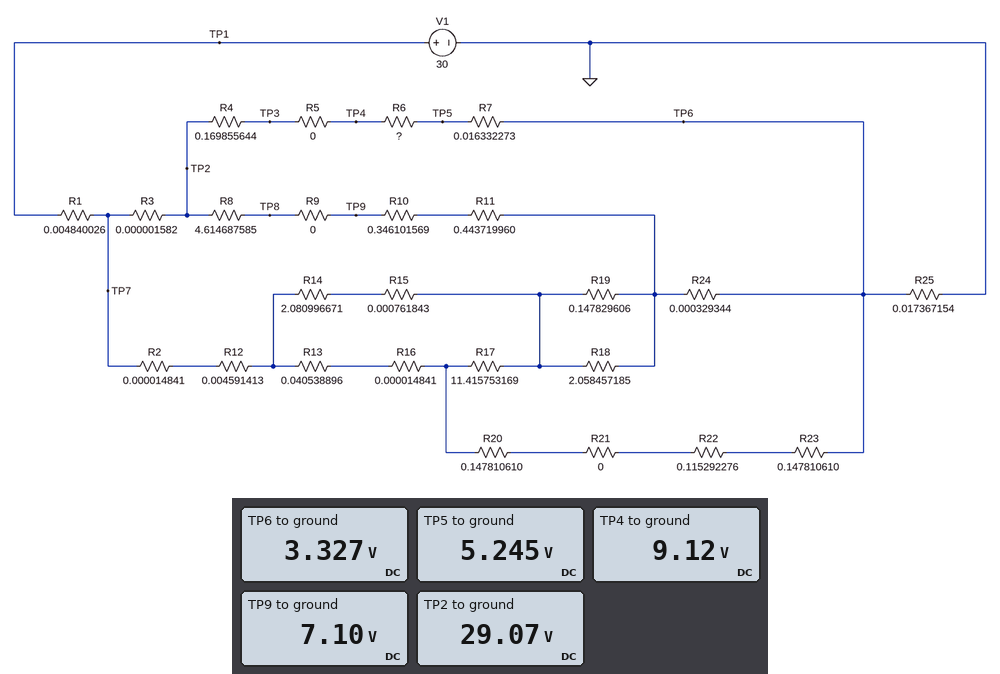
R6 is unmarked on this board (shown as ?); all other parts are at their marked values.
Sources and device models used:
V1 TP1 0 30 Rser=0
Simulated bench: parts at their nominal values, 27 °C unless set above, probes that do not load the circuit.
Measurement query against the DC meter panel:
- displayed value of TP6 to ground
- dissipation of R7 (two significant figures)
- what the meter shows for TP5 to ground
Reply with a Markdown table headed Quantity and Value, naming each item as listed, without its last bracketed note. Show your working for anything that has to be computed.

| Quantity | Value |
|---|---|
| displayed value of TP6 to ground | 3.327 V |
| dissipation of R7 | (5.245 V - 3.327 V)^2 / 16.33 mΩ = 230 W |
| what the meter shows for TP5 to ground | 5.245 V |
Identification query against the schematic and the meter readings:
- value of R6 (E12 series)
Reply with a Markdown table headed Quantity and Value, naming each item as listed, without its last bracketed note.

| Quantity | Value |
|---|---|
| value of R6 | 0.033 Ω |
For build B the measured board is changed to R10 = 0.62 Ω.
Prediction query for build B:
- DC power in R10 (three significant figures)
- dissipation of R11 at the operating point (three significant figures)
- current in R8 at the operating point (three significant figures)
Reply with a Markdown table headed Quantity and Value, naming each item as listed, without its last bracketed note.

| Quantity | Value |
|---|---|
| DC power in R10 | 12.7 W |
| dissipation of R11 at the operating point | 9.12 W |
| current in R8 at the operating point | 4.53 A |
